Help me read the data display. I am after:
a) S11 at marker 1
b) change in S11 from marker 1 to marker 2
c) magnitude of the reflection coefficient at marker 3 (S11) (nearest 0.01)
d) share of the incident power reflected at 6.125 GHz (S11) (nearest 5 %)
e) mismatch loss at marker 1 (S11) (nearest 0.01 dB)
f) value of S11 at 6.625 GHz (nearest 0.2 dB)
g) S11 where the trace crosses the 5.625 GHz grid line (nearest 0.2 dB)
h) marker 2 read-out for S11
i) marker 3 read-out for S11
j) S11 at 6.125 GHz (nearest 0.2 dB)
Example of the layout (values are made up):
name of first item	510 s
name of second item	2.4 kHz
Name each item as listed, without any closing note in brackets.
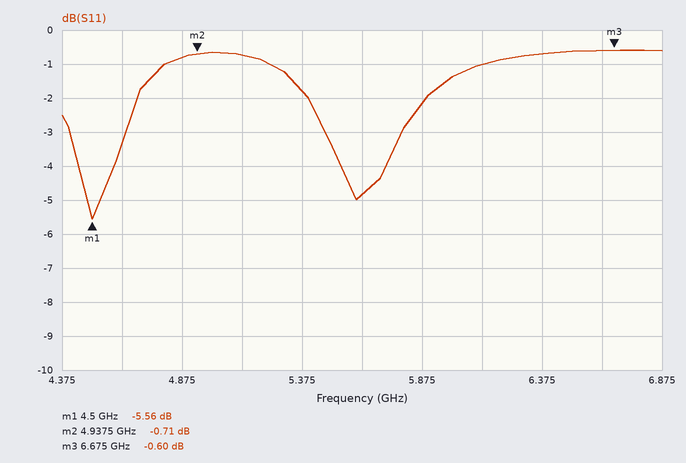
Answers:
S11 at marker 1	-5.56 dB
change in S11 from marker 1 to marker 2	4.85 dB
magnitude of the reflection coefficient at marker 3 (S11)	0.93
share of the incident power reflected at 6.125 GHz (S11)	80 %
mismatch loss at marker 1 (S11)	1.41 dB
value of S11 at 6.625 GHz	-0.6 dB
S11 where the trace crosses the 5.625 GHz grid line	-4.8 dB
marker 2 read-out for S11	-0.71 dB
marker 3 read-out for S11	-0.60 dB
S11 at 6.125 GHz	-1.0 dB
